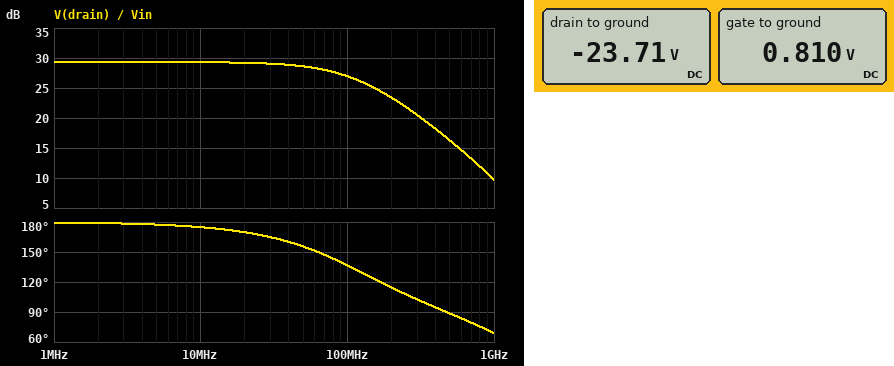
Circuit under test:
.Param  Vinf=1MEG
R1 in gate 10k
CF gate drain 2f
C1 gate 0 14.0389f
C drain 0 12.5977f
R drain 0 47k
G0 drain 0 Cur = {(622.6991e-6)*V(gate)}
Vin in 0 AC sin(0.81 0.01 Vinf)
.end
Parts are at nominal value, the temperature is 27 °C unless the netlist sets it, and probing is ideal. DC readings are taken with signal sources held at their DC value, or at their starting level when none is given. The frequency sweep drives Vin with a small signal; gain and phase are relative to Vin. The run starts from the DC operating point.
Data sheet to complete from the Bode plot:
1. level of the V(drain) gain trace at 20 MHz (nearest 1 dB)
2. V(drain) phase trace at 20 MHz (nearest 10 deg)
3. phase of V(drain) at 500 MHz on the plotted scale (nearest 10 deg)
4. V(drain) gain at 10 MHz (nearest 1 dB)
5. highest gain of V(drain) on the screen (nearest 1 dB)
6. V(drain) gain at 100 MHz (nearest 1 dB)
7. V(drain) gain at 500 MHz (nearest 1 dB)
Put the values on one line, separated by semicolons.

29 dB; 170 deg; 90 deg; 29 dB; 29 dB; 27 dB; 16 dB
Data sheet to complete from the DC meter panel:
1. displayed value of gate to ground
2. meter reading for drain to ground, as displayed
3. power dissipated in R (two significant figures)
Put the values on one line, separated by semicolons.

0.810 V; -23.71 V; 12 mW
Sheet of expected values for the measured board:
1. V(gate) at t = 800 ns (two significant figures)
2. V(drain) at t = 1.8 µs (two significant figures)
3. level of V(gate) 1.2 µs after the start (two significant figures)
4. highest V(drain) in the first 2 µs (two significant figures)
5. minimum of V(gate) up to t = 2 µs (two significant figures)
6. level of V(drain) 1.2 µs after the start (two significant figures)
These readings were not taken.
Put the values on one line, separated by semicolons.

800 mV; -23 V; 820 mV; -23 V; 800 mV; -24 V
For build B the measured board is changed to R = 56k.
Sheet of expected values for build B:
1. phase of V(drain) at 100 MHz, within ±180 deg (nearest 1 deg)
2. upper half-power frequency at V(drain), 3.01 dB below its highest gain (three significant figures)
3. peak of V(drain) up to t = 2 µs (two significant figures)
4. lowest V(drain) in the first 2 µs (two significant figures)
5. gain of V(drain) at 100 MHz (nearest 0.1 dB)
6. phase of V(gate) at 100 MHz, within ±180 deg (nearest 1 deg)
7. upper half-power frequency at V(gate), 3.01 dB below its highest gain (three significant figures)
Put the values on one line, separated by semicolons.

132 deg; 99.6 MHz; -28 V; -29 V; 27.8 dB; -21 deg; 144 MHz
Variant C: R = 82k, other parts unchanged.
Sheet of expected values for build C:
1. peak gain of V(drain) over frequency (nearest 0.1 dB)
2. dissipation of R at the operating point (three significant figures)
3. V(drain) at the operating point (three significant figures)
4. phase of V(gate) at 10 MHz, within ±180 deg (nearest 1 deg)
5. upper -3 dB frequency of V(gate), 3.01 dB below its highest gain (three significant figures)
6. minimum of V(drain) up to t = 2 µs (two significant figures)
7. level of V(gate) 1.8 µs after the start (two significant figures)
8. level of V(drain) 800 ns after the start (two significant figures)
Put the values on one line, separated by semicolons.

34.2 dB; 20.9 mW; -41.4 V; -4 deg; 102 MHz; -42 V; 800 mV; -41 V
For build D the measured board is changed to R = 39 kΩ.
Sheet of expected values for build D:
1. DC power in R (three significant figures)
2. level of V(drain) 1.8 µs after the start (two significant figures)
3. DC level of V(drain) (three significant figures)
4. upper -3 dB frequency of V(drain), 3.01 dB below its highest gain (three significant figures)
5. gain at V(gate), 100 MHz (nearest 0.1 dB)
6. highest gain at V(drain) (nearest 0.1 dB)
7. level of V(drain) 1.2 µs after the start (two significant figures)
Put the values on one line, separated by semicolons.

9.92 mW; -19 V; -19.7 V; 139 MHz; -1.3 dB; 27.7 dB; -20 V
